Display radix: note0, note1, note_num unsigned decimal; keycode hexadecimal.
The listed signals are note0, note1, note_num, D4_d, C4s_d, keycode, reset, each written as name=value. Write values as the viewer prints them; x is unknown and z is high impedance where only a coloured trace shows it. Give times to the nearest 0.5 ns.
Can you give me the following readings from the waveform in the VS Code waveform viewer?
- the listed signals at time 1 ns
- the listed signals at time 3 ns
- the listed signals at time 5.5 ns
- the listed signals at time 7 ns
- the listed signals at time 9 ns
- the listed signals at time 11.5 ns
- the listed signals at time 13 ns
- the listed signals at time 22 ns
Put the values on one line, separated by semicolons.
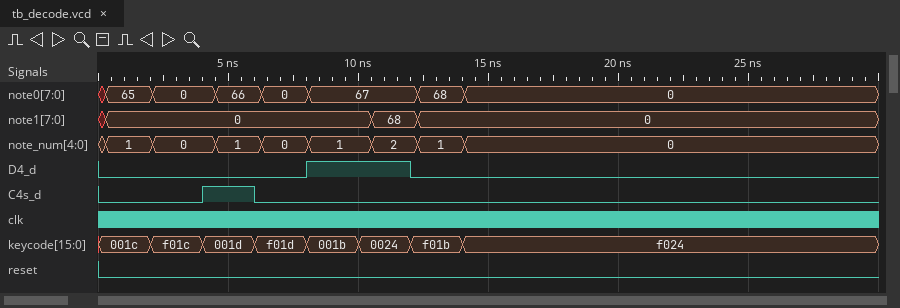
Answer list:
note0=65, note1=0, note_num=1, D4_d=0, C4s_d=0, keycode=001c, reset=0; note0=0, note1=0, note_num=0, D4_d=0, C4s_d=0, keycode=f01c, reset=0; note0=66, note1=0, note_num=1, D4_d=0, C4s_d=1, keycode=001d, reset=0; note0=0, note1=0, note_num=0, D4_d=0, C4s_d=0, keycode=f01d, reset=0; note0=67, note1=0, note_num=1, D4_d=1, C4s_d=0, keycode=001b, reset=0; note0=67, note1=68, note_num=2, D4_d=1, C4s_d=0, keycode=0024, reset=0; note0=68, note1=0, note_num=1, D4_d=0, C4s_d=0, keycode=f01b, reset=0; note0=0, note1=0, note_num=0, D4_d=0, C4s_d=0, keycode=f024, reset=0
